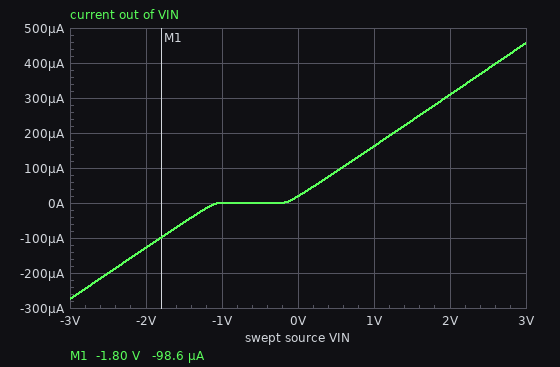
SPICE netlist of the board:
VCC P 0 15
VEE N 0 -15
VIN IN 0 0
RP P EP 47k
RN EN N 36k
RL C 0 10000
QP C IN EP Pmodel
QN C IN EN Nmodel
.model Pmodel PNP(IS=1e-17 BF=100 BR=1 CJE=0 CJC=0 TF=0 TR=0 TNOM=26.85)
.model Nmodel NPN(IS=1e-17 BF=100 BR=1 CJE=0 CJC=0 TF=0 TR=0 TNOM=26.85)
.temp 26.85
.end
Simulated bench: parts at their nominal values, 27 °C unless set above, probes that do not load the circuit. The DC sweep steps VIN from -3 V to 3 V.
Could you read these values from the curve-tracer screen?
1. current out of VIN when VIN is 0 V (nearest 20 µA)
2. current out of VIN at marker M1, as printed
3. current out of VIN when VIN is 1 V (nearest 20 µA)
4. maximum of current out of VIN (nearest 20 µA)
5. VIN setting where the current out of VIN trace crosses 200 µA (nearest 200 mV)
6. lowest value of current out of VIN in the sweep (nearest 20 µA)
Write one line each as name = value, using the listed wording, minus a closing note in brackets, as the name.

current out of VIN when VIN is 0 V = 20 µA
current out of VIN at marker M1, as printed = -98.6 µA
current out of VIN when VIN is 1 V = 160 µA
maximum of current out of VIN = 460 µA
VIN setting where the current out of VIN trace crosses 200 µA = 1.2 V
lowest value of current out of VIN in the sweep = -280 µA
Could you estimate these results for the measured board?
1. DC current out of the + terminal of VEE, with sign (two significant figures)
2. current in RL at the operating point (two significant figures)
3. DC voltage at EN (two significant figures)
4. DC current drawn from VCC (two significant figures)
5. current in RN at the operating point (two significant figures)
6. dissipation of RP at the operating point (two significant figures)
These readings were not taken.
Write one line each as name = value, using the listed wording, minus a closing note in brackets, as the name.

DC current out of the + terminal of VEE, with sign = -390 µA
current in RL at the operating point = 73 µA
DC voltage at EN = -810 mV
DC current drawn from VCC = 300 µA
current in RN at the operating point = 390 µA
dissipation of RP at the operating point = 4.3 mW
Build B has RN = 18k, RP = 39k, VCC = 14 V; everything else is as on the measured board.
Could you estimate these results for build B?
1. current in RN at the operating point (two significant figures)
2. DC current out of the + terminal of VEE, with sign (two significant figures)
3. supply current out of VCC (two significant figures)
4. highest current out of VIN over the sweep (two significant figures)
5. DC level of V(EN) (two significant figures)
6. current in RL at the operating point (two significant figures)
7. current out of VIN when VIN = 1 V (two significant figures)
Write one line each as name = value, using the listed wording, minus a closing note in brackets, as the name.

current in RN at the operating point = 790 µA
DC current out of the + terminal of VEE, with sign = -790 µA
supply current out of VCC = 340 µA
highest current out of VIN over the sweep = 910 µA
DC level of V(EN) = -840 mV
current in RL at the operating point = 81 µA
current out of VIN when VIN = 1 V = 550 µA
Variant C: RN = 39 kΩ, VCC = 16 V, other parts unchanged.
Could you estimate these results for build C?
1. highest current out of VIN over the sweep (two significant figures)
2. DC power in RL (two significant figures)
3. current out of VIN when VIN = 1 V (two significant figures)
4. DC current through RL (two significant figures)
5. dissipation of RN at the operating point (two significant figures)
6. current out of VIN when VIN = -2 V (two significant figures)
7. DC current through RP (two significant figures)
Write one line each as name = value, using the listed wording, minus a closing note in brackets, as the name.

highest current out of VIN over the sweep = 400 µA
DC power in RL = 16 µW
current out of VIN when VIN = 1 V = 110 µA
DC current through RL = 40 µA
dissipation of RN at the operating point = 5.2 mW
current out of VIN when VIN = -2 V = -170 µA
DC current through RP = 320 µA
